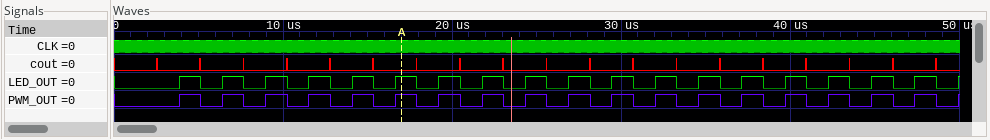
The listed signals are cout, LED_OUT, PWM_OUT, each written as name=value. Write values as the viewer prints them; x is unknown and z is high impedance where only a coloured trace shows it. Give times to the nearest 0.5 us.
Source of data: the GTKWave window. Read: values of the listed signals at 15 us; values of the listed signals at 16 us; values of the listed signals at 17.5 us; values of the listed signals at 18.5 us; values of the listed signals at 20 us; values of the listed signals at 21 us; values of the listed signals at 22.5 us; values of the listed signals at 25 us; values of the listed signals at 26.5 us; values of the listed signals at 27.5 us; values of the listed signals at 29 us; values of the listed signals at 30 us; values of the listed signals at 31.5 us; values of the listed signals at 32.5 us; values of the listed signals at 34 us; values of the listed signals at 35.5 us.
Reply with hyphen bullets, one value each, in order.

- cout=0, LED_OUT=1, PWM_OUT=1
- cout=0, LED_OUT=0, PWM_OUT=0
- cout=0, LED_OUT=1, PWM_OUT=1
- cout=0, LED_OUT=0, PWM_OUT=0
- cout=0, LED_OUT=1, PWM_OUT=1
- cout=0, LED_OUT=0, PWM_OUT=0
- cout=0, LED_OUT=1, PWM_OUT=1
- cout=0, LED_OUT=1, PWM_OUT=1
- cout=0, LED_OUT=0, PWM_OUT=0
- cout=0, LED_OUT=1, PWM_OUT=1
- cout=0, LED_OUT=0, PWM_OUT=0
- cout=0, LED_OUT=1, PWM_OUT=1
- cout=0, LED_OUT=0, PWM_OUT=0
- cout=0, LED_OUT=1, PWM_OUT=1
- cout=0, LED_OUT=0, PWM_OUT=0
- cout=0, LED_OUT=1, PWM_OUT=1
